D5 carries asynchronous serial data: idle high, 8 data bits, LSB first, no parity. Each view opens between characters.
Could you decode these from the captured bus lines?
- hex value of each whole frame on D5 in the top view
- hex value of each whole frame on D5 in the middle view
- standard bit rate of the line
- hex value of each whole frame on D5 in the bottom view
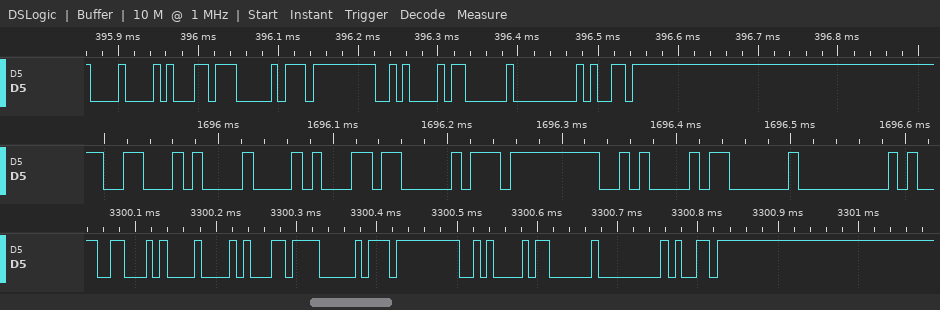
08, B1, D0, FF, 0A, 03, 00, D9
46, 08, B1, D0, FF, 0A, 03, 00
115200 baud
46, 08, B1, D0, FF, 0A, 03, 00, D9
